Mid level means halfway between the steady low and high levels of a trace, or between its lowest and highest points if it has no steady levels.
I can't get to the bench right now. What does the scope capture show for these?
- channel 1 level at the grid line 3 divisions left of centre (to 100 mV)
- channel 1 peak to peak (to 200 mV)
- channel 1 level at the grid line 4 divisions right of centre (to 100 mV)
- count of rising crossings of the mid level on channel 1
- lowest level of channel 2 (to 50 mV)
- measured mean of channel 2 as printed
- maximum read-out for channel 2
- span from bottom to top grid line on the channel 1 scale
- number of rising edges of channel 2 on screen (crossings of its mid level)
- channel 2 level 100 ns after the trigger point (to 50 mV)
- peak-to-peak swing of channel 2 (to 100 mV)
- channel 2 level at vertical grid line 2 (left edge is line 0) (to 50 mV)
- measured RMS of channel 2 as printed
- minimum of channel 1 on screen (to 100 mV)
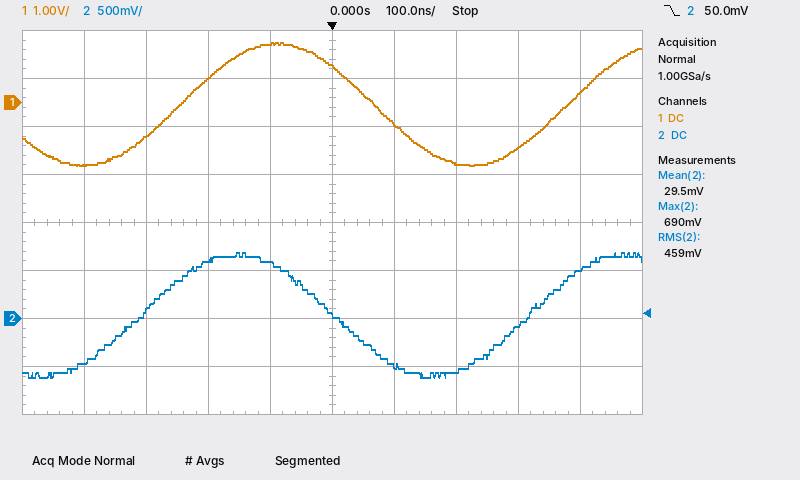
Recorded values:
-700 mV
2.6 V
200 mV
2
-600 mV
29.5 mV
690 mV
8 V
2
-500 mV
1.30 V
50 mV
459 mV
-1.3 V
